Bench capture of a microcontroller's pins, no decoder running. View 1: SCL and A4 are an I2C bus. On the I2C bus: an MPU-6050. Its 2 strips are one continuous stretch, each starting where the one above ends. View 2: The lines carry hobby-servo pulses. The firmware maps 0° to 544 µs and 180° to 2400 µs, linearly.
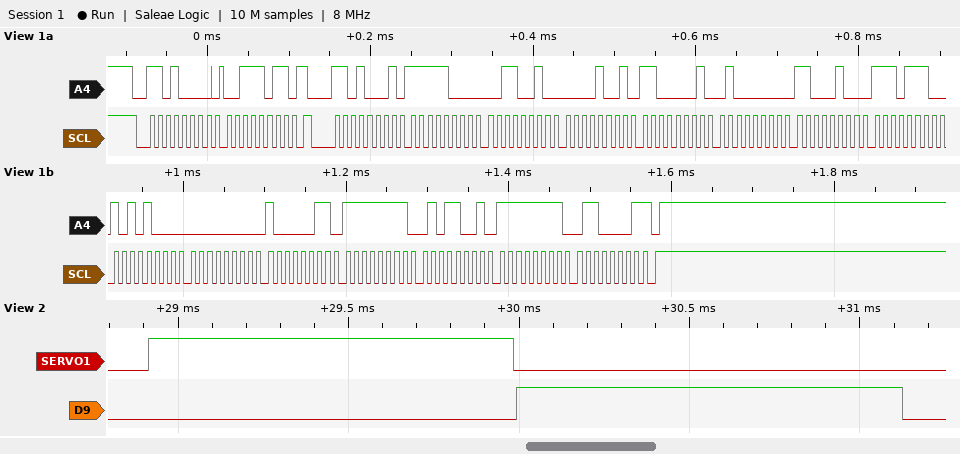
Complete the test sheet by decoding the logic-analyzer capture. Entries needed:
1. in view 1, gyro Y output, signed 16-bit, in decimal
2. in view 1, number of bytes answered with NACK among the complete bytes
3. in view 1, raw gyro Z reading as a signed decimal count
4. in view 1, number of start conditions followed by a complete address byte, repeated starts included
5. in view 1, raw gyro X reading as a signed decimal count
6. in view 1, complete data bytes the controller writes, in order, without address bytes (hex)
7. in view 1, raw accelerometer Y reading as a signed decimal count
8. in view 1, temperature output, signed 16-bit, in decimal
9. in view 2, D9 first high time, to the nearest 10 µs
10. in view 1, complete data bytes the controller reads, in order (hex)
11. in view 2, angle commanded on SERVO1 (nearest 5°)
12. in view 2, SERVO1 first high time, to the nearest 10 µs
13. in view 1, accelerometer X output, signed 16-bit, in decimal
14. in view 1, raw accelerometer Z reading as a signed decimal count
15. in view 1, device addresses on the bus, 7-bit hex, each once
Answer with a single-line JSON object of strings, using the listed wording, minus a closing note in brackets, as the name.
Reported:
{"in view 1, gyro Y output, signed 16-bit, in decimal": "-167", "in view 1, number of bytes answered with NACK among the complete bytes": "1", "in view 1, raw gyro Z reading as a signed decimal count": "-159", "in view 1, number of start conditions followed by a complete address byte, repeated starts included": "2", "in view 1, raw gyro X reading as a signed decimal count": "131", "in view 1, complete data bytes the controller writes, in order, without address bytes": "3B", "in view 1, raw accelerometer Y reading as a signed decimal count": "2497", "in view 1, temperature output, signed 16-bit, in decimal": "-4440", "in view 2, D9 first high time, to the nearest 10 µs": "1130 µs", "in view 1, complete data bytes the controller reads, in order": "F8 32 09 C1 40 C4 EE A8 00 83 FF 59 FF 61", "in view 2, angle commanded on SERVO1": "50°", "in view 2, SERVO1 first high time, to the nearest 10 µs": "1070 µs", "in view 1, accelerometer X output, signed 16-bit, in decimal": "-1998", "in view 1, raw accelerometer Z reading as a signed decimal count": "16580", "in view 1, device addresses on the bus, 7-bit hex, each once": "0x68"}
